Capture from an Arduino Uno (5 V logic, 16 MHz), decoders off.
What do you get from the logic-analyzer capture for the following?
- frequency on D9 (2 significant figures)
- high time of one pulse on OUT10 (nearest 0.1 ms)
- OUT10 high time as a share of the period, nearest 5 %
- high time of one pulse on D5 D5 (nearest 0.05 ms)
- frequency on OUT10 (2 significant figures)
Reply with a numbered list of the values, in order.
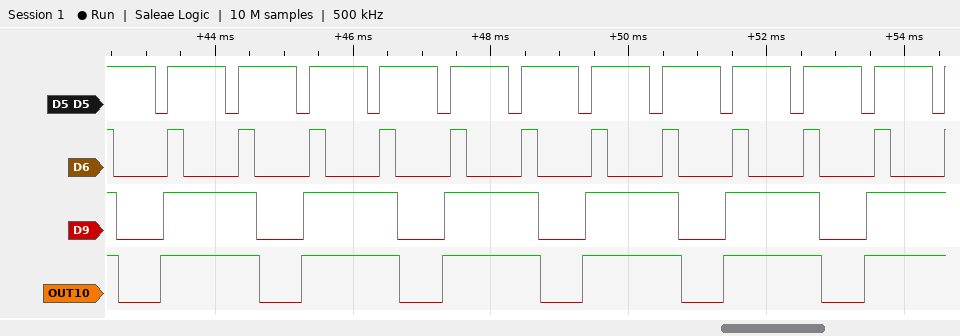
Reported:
1. 490 Hz
2. 1.4 ms
3. 70 %
4. 0.85 ms
5. 490 Hz
